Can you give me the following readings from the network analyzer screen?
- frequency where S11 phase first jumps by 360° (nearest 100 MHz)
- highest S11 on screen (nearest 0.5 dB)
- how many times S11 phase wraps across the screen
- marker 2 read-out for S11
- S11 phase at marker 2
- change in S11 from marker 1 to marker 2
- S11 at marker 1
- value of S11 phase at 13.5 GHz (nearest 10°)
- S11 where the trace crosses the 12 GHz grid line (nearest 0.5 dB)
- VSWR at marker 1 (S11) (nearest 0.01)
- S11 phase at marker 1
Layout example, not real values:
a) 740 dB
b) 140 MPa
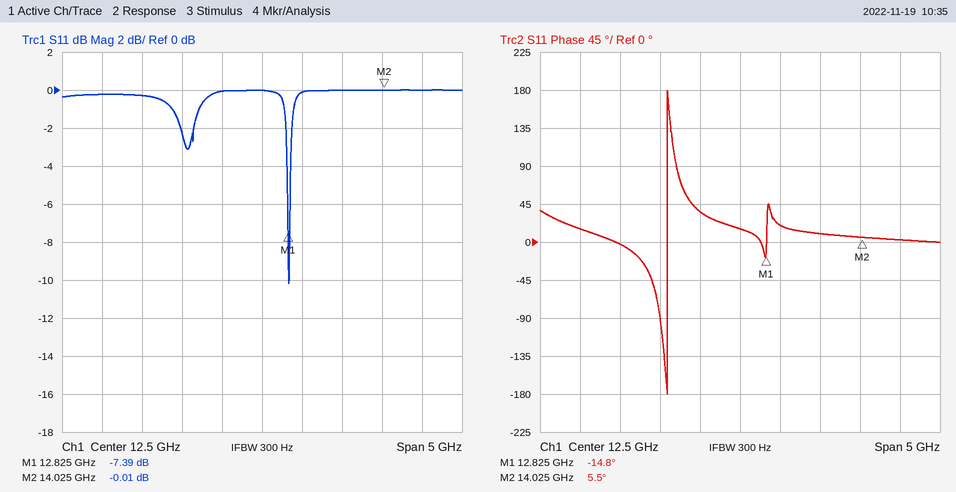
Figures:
a) 11.6 GHz
b) 0.0 dB
c) 1
d) -0.01 dB
e) 5.5°
f) 7.38 dB
g) -7.39 dB
h) 10°
i) 0.0 dB
j) 2.49
k) -14.8°
